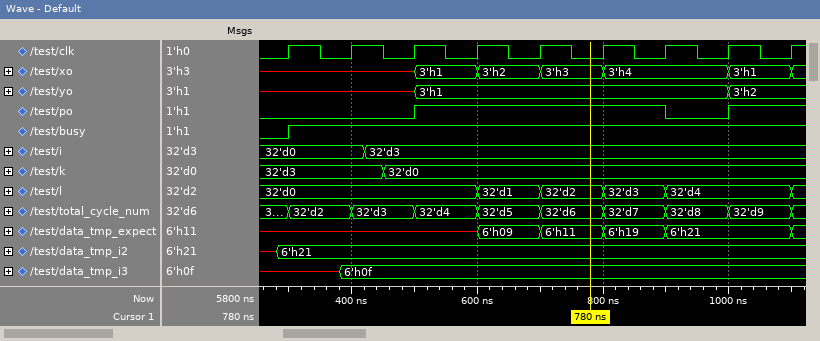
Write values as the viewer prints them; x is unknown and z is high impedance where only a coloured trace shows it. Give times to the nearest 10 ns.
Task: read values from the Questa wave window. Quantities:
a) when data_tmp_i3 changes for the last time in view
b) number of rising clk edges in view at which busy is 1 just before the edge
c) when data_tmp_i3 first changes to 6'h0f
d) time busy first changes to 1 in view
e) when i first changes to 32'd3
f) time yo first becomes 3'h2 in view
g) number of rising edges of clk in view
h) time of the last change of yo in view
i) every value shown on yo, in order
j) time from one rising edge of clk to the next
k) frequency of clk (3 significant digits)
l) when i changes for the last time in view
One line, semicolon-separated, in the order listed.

380 ns; 8; 380 ns; 300 ns; 420 ns; 1000 ns; 9; 1000 ns; x, 3'h1, 3'h2; 100 ns; 10.0 MHz; 420 ns
